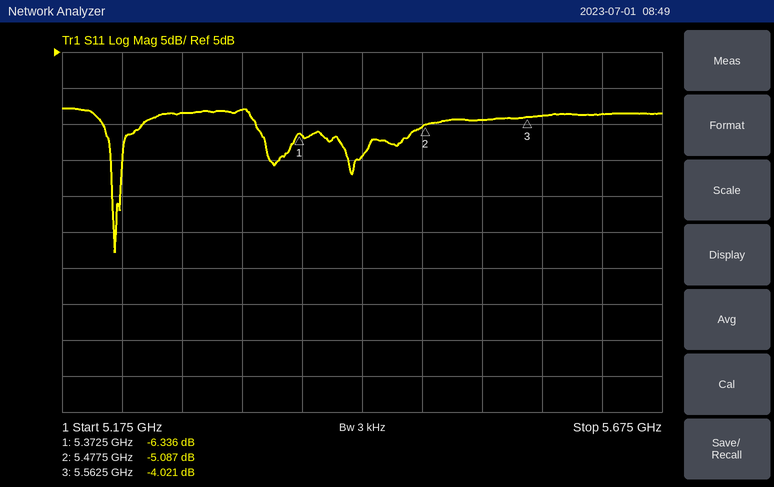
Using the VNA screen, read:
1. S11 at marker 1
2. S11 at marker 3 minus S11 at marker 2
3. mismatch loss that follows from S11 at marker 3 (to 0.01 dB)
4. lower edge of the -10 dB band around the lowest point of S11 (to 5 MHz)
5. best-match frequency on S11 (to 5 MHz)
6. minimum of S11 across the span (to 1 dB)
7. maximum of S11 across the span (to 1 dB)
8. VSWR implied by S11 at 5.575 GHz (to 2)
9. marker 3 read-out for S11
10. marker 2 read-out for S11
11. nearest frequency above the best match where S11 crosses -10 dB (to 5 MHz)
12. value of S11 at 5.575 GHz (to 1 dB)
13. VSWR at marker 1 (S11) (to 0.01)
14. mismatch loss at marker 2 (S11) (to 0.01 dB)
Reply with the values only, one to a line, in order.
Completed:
-6.336 dB
1.066 dB
2.19 dB
5.215 GHz
5.220 GHz
-23 dB
-3 dB
4
-4.021 dB
-5.087 dB
5.225 GHz
-4 dB
2.86
1.61 dB
